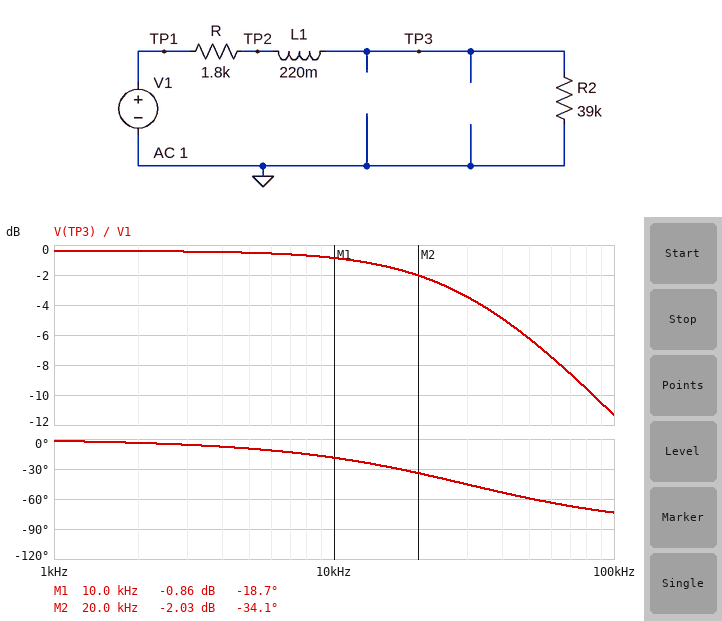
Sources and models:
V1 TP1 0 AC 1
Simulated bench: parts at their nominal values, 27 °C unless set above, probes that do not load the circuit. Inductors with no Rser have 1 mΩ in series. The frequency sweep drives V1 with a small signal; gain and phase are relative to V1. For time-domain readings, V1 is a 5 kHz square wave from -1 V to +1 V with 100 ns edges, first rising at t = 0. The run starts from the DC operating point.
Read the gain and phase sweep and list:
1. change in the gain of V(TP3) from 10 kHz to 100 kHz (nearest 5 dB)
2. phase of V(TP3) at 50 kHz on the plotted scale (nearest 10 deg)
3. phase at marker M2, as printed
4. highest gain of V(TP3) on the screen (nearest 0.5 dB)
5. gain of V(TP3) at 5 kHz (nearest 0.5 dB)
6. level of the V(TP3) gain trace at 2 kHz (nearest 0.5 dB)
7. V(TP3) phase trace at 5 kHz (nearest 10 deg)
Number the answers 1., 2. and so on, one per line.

1. -10 dB
2. -60 deg
3. -34.1 deg
4. -0.5 dB
5. -0.5 dB
6. -0.5 dB
7. -10 deg
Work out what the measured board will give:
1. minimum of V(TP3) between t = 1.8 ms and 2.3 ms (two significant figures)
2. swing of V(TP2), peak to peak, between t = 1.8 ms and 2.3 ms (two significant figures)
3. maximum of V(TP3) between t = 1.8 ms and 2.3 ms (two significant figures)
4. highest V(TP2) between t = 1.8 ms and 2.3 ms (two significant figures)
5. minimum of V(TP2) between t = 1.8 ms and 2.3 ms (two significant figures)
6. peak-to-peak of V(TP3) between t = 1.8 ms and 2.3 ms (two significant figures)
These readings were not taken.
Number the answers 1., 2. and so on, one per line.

1. -960 mV
2. 2.1 V
3. 960 mV
4. 1.0 V
5. -1.0 V
6. 1.9 V
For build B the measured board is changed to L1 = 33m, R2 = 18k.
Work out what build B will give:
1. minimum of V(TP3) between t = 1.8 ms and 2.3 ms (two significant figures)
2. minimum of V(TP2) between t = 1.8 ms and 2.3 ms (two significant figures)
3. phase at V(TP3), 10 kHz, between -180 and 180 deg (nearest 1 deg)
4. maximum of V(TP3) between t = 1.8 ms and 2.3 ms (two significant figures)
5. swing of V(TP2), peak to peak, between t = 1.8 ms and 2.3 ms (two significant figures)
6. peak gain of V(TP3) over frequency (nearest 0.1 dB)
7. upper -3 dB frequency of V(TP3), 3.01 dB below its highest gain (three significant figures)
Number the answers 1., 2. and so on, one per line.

1. -910 mV
2. -1.1 V
3. -6 deg
4. 910 mV
5. 2.2 V
6. -0.8 dB
7. 95.5 kHz
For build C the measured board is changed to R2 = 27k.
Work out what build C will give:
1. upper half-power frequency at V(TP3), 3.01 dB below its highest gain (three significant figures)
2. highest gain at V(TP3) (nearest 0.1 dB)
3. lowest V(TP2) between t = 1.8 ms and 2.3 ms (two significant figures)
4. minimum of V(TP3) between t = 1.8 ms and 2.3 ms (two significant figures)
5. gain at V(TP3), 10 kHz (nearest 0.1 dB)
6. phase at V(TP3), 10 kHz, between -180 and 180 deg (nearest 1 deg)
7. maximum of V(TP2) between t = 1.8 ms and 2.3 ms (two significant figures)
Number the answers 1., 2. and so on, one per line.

1. 20.8 kHz
2. -0.6 dB
3. -1.1 V
4. -940 mV
5. -1.5 dB
6. -26 deg
7. 1.1 V
